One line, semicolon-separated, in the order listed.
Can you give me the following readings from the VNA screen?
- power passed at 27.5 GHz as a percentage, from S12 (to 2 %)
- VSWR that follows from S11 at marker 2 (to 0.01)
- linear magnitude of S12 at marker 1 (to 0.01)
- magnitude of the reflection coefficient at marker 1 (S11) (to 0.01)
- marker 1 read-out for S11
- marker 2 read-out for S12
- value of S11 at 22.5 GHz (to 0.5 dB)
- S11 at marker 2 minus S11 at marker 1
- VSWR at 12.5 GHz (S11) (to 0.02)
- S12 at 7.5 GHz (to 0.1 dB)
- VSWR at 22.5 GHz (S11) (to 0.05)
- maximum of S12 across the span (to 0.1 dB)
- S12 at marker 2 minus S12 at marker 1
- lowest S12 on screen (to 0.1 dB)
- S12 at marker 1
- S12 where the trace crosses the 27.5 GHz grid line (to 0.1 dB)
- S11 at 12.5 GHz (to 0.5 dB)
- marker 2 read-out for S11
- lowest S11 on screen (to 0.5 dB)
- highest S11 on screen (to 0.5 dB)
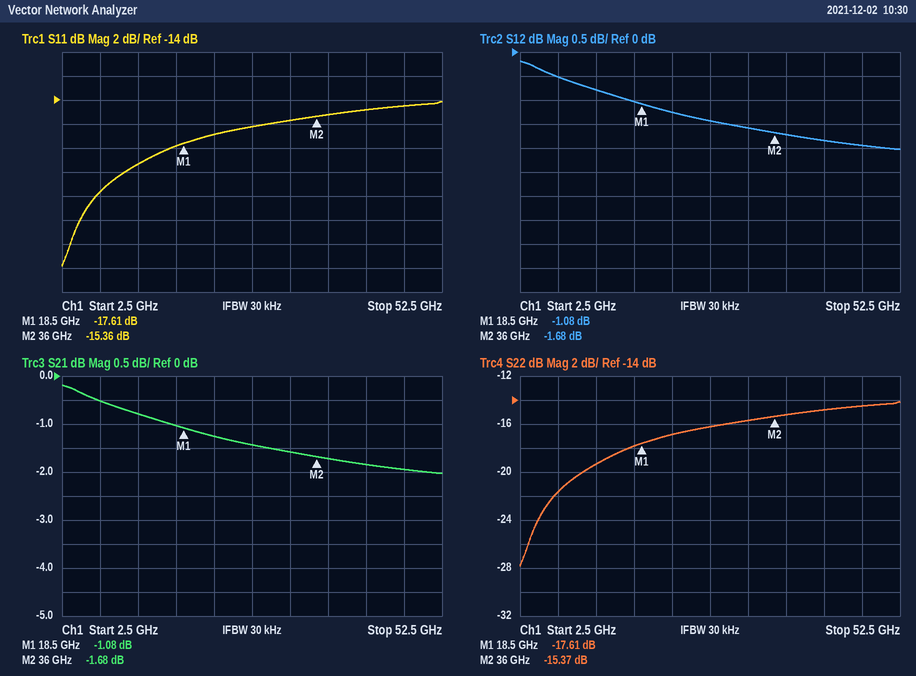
72 %; 1.41; 0.88; 0.13; -17.61 dB; -1.68 dB; -17.0 dB; 2.25 dB; 1.24; -0.5 dB; 1.35; -0.2 dB; -0.60 dB; -2.0 dB; -1.08 dB; -1.4 dB; -19.5 dB; -15.36 dB; -28.0 dB; -14.0 dB
